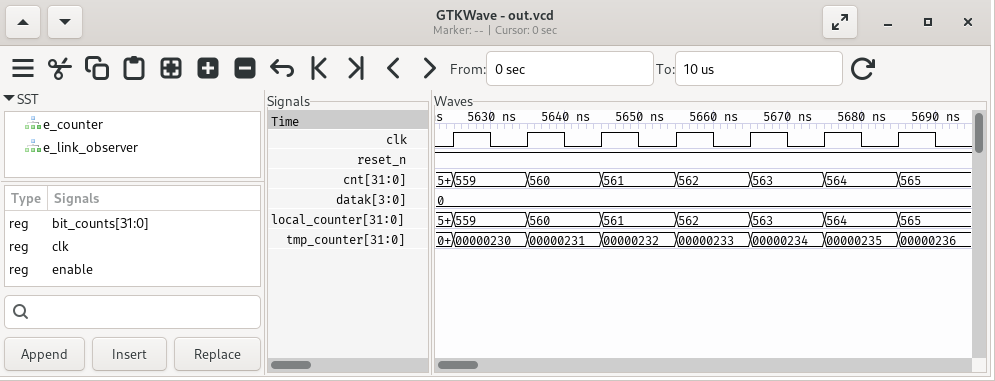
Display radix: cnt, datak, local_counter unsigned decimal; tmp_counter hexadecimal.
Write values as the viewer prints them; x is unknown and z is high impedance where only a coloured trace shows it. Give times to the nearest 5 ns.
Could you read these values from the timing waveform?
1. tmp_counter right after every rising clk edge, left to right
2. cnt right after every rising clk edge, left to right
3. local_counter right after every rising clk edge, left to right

00000230, 00000231, 00000232, 00000233, 00000234, 00000235, 00000236
559, 560, 561, 562, 563, 564, 565
559, 560, 561, 562, 563, 564, 565
